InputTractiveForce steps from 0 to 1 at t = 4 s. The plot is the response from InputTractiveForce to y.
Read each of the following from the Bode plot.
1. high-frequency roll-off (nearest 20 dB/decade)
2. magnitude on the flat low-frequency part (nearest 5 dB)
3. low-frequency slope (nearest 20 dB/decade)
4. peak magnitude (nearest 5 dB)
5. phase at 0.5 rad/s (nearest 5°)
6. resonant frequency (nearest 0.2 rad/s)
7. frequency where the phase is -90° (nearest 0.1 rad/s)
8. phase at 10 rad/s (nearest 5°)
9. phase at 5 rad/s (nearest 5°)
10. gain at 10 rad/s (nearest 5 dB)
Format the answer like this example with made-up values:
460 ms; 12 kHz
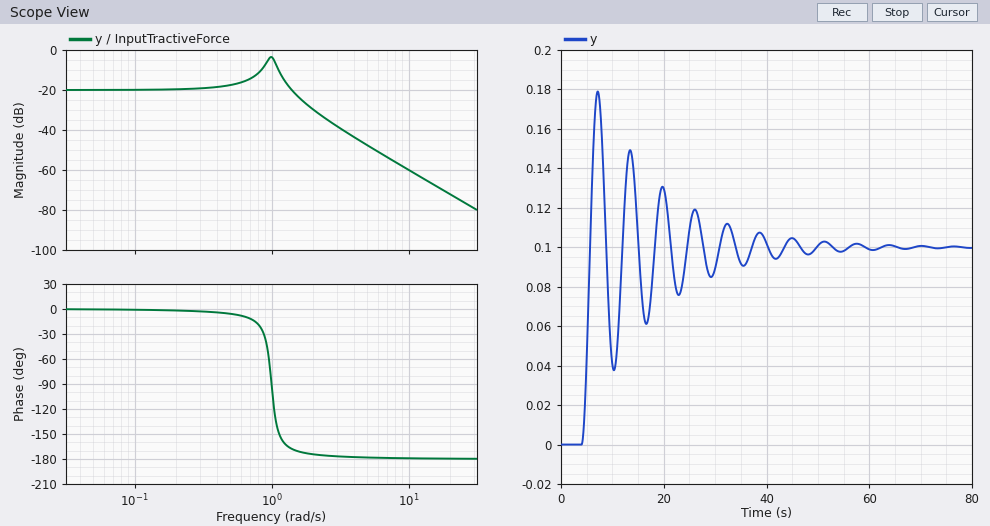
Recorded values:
-40 dB/decade; -20 dB; 0 dB/decade; -5 dB; -5°; 1.0 rad/s; 1.0 rad/s; -180°; -180°; -60 dB
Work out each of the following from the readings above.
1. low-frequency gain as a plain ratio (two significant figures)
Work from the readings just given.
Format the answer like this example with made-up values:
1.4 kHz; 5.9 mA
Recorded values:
0.10
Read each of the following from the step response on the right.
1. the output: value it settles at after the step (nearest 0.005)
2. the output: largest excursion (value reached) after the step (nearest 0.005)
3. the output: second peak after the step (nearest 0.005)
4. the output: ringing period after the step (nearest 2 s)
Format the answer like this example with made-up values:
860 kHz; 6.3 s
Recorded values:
0.100; 0.180; 0.150; 6 s
